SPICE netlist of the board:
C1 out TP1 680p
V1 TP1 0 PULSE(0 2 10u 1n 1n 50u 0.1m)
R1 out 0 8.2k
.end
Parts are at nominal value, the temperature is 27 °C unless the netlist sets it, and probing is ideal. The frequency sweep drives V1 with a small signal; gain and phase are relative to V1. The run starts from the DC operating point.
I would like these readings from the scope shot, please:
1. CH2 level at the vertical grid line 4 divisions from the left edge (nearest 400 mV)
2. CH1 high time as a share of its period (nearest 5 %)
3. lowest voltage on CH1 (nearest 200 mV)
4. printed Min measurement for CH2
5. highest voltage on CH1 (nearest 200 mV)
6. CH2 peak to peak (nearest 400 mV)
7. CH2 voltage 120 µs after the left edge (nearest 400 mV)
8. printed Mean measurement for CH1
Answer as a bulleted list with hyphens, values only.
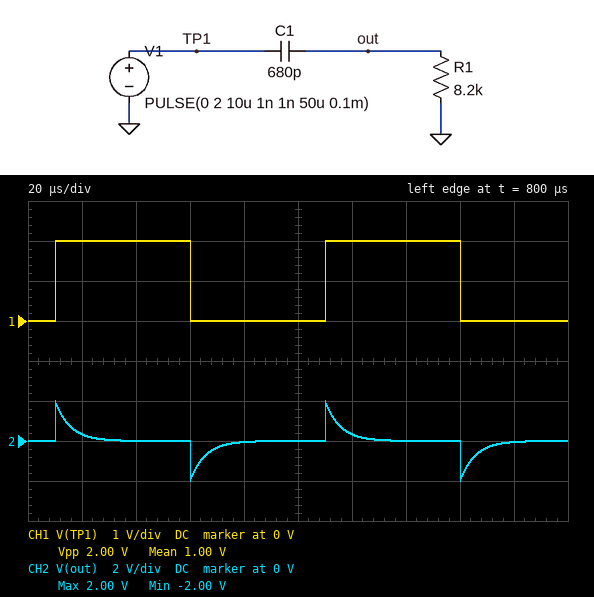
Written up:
- 0 V
- 50 %
- 0 V
- -2.00 V
- 2.0 V
- 4.0 V
- 400 mV
- 1.00 V
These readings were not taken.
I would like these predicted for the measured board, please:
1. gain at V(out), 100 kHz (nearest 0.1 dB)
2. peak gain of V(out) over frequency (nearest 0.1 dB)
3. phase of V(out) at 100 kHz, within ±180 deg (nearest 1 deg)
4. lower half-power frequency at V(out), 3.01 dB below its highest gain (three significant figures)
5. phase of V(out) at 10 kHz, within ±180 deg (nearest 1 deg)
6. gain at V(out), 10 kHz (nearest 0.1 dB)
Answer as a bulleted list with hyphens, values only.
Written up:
- -0.3 dB
- 0 dB
- 16 deg
- 28.5 kHz
- 71 deg
- -9.6 dB
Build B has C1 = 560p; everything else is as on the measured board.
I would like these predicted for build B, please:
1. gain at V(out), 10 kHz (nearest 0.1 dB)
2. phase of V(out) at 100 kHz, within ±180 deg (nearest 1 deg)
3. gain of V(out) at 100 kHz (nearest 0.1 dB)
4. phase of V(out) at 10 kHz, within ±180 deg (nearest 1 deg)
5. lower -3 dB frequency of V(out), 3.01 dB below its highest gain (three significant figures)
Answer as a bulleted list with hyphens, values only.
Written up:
- -11.1 dB
- 19 deg
- -0.5 dB
- 74 deg
- 34.7 kHz
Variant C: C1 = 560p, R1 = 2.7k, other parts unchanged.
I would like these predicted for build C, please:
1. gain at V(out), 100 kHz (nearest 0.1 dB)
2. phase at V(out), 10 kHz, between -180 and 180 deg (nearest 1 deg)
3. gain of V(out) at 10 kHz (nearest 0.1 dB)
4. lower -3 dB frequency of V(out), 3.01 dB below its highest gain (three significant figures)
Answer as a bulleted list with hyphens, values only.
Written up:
- -3.2 dB
- 85 deg
- -20.5 dB
- 105 kHz
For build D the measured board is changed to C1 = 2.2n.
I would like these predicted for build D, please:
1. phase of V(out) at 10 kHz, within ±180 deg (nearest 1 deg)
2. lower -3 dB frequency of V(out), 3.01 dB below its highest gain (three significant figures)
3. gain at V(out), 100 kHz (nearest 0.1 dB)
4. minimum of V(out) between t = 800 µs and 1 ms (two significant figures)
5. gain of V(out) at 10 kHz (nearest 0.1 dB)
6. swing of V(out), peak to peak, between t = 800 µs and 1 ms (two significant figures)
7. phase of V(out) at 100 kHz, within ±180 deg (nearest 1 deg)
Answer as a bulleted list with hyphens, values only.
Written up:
- 41 deg
- 8.82 kHz
- 0 dB
- -1.9 V
- -2.5 dB
- 3.8 V
- 5 deg
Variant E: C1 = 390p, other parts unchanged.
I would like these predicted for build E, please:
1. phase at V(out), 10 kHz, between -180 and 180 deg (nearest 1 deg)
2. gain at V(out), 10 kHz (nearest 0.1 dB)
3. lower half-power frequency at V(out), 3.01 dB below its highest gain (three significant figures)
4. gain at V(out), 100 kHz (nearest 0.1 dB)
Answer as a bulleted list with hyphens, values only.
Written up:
- 79 deg
- -14.1 dB
- 49.8 kHz
- -1.0 dB
